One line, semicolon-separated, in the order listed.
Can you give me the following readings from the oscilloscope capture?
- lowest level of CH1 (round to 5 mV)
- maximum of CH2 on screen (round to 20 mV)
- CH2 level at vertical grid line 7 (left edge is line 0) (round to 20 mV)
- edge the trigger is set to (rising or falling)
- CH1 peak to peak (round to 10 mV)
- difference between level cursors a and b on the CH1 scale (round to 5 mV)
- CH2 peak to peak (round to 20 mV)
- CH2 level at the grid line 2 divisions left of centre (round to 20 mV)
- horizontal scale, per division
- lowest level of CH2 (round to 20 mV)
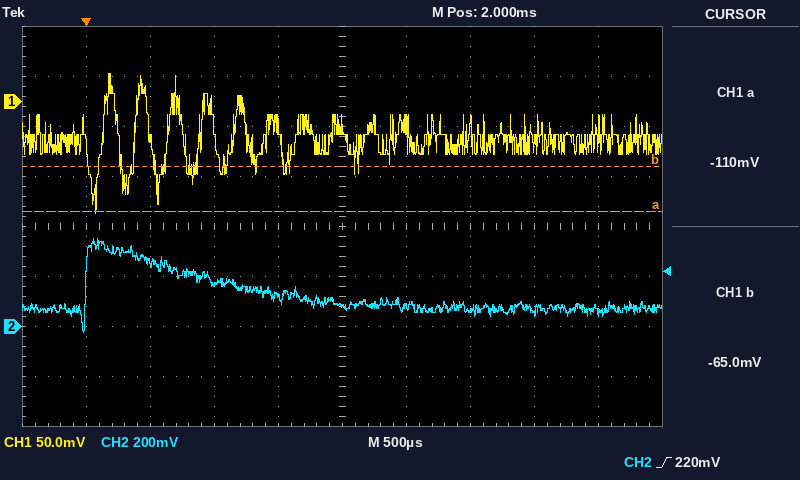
-110 mV; 360 mV; 60 mV; rising; 140 mV; 45 mV; 380 mV; 160 mV; 500 µs; -20 mV
